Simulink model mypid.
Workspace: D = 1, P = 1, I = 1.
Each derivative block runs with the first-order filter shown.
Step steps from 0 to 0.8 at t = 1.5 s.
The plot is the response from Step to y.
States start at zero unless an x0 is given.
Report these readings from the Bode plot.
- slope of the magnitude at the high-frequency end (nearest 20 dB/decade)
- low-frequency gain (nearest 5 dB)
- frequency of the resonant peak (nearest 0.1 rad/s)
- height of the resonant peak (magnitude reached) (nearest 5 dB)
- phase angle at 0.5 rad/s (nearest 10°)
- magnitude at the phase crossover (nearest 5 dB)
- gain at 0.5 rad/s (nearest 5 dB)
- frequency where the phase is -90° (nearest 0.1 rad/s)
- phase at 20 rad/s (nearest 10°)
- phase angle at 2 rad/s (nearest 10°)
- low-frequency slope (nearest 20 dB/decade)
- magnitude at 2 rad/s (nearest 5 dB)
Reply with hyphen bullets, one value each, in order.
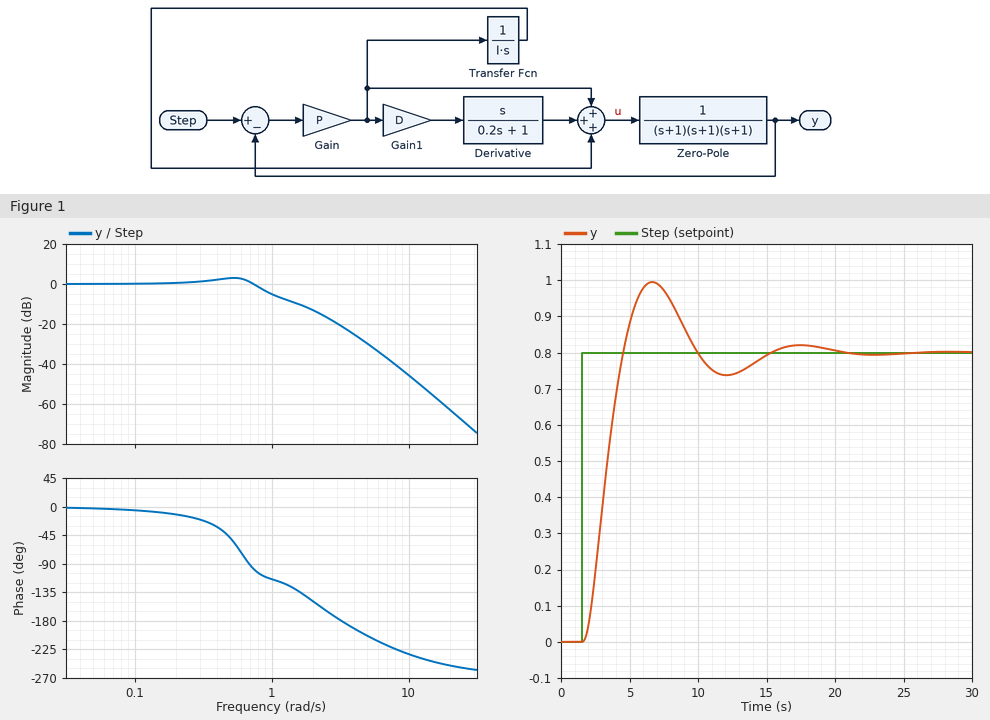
- -60 dB/decade
- 0 dB
- 0.5 rad/s
- 5 dB
- -50°
- -20 dB
- 5 dB
- 0.7 rad/s
- -250°
- -150°
- 0 dB/decade
- -15 dB
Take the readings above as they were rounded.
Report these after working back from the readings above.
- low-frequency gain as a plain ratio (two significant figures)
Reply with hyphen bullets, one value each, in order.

- 1.0
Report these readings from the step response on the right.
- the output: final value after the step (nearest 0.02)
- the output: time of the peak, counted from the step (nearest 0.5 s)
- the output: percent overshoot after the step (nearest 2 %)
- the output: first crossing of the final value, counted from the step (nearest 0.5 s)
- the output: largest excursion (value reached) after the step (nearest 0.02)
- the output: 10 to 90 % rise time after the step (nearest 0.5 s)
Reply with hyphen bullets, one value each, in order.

- 0.80
- 5.0 s
- 24 %
- 3.0 s
- 1.00
- 2.0 s
